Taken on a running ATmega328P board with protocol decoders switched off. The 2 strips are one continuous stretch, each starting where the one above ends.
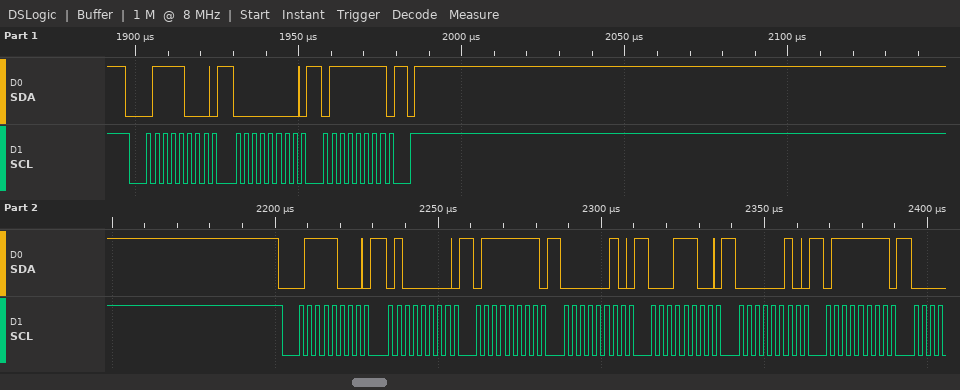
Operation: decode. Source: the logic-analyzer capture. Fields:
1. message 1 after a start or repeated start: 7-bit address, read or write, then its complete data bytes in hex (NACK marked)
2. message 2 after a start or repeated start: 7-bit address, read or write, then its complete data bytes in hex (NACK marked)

0x3C write: 00 7F
0x3C write: 40 7F 02 1C 02 7F
